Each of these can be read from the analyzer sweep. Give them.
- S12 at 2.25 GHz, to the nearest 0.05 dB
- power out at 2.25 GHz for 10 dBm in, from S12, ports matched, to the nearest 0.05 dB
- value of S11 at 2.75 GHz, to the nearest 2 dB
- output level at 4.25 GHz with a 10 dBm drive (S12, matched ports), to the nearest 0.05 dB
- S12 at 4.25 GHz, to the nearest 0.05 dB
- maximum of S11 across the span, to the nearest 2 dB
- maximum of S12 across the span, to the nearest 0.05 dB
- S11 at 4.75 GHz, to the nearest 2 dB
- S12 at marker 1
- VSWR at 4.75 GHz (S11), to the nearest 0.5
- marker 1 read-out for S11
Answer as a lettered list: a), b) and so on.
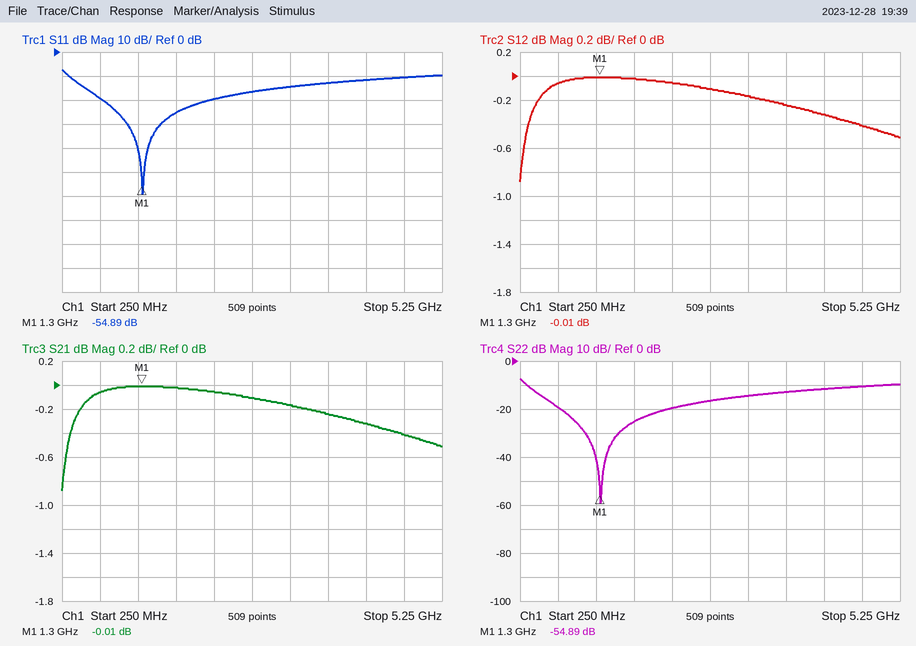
a) -0.05 dB
b) 9.95 dBm
c) -16 dB
d) 9.70 dBm
e) -0.30 dB
f) -8 dB
g) 0.00 dB
h) -10 dB
i) -0.01 dB
j) 2.0
k) -54.89 dB
